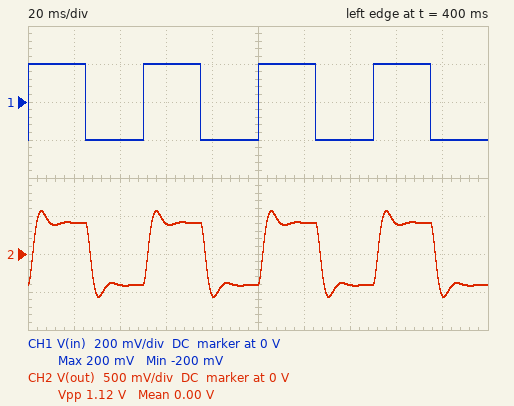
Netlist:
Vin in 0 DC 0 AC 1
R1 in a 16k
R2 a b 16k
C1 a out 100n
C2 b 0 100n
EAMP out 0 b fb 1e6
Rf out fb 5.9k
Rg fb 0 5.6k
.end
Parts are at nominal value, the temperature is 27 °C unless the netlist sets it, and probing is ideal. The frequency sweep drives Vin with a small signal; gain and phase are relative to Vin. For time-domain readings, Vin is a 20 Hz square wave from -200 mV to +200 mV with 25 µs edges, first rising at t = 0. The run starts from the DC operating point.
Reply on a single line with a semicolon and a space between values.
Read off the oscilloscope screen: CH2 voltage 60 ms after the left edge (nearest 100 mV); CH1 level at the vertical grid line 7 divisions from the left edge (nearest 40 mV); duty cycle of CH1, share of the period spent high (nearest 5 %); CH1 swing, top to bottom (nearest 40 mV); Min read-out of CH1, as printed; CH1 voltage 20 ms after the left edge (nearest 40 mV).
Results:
400 mV; -200 mV; 50 %; 400 mV; -200 mV; 200 mV
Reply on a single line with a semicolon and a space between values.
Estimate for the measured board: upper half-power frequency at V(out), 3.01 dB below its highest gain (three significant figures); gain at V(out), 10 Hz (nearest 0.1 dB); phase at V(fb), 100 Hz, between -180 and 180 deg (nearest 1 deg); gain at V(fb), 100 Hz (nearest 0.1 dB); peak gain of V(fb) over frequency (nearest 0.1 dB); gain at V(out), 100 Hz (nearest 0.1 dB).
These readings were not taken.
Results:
117 Hz; 6.3 dB; -91 deg; 0.4 dB; 1.6 dB; 6.7 dB
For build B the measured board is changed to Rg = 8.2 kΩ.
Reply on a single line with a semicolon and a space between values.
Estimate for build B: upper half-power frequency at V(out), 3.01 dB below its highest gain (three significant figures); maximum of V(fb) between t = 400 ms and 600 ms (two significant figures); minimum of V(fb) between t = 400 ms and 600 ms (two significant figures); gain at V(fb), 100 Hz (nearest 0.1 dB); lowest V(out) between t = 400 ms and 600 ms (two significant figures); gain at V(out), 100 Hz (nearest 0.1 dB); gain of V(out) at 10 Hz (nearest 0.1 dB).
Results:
107 Hz; 230 mV; -230 mV; -2.2 dB; -390 mV; 2.5 dB; 4.7 dB
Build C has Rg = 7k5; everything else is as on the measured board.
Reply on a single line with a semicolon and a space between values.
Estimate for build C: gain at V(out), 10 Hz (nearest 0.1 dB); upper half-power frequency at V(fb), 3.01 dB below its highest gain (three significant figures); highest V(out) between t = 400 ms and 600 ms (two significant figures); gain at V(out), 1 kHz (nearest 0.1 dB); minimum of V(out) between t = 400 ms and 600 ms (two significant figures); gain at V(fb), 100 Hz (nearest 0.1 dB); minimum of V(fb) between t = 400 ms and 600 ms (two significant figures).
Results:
5.1 dB; 110 Hz; 420 mV; -35.0 dB; -420 mV; -1.7 dB; -240 mV
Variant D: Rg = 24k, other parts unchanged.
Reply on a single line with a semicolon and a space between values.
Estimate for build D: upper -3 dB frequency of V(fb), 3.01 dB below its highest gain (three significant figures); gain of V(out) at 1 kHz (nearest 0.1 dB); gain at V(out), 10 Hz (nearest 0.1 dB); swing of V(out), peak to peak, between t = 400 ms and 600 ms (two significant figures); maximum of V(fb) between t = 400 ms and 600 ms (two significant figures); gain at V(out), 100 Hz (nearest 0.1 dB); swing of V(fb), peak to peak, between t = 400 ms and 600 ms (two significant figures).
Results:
76.9 Hz; -38.2 dB; 1.9 dB; 500 mV; 200 mV; -3.0 dB; 400 mV
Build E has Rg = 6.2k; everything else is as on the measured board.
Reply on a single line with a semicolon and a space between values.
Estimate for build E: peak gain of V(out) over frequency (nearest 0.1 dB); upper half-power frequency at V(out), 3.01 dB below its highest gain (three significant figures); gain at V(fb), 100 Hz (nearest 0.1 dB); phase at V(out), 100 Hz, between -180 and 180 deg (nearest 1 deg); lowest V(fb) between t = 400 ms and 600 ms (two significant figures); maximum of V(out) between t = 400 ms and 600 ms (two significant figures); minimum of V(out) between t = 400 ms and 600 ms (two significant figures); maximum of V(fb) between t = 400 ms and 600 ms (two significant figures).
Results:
6.8 dB; 115 Hz; -0.5 dB; -91 deg; -260 mV; 500 mV; -500 mV; 260 mV
